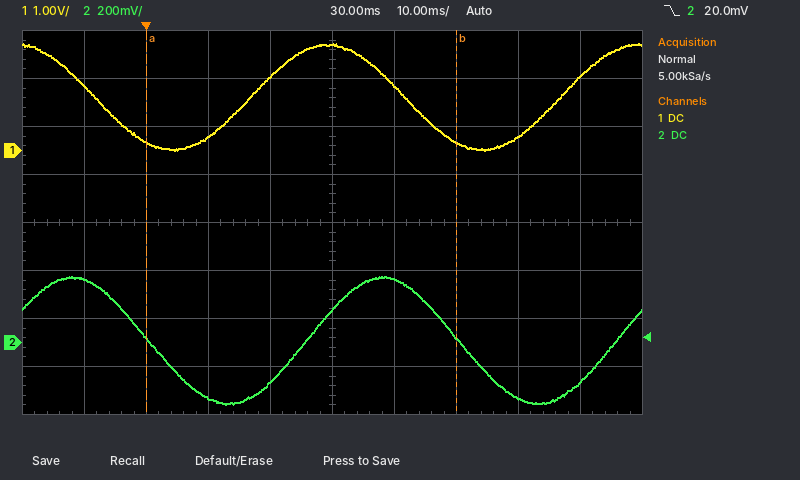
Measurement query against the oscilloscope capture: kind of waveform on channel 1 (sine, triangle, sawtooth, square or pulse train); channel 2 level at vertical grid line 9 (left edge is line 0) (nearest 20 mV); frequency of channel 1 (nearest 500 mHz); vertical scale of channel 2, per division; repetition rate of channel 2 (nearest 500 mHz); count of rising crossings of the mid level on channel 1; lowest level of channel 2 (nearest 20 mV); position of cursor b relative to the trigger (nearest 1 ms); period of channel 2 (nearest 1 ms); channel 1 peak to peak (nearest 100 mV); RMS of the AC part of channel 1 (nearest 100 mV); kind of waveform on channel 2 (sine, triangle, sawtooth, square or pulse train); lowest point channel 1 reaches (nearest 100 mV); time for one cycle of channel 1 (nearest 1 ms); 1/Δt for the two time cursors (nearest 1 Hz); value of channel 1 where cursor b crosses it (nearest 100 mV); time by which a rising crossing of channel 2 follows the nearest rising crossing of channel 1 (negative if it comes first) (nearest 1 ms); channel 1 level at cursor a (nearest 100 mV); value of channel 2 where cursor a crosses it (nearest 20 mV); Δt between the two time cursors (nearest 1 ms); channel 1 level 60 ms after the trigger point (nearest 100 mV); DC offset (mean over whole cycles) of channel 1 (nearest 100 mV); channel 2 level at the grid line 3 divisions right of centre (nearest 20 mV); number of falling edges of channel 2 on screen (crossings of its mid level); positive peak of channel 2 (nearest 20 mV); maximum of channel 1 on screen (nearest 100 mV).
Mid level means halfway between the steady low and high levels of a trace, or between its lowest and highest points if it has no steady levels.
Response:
sine
-160 mV
20.0 Hz
200 mV
20.0 Hz
2
-260 mV
+50 ms
50 ms
2.2 V
800 mV
sine
0.0 V
50 ms
20 Hz
200 mV
+9 ms
200 mV
20 mV
50 ms
300 mV
1.1 V
-240 mV
2
280 mV
2.2 V
